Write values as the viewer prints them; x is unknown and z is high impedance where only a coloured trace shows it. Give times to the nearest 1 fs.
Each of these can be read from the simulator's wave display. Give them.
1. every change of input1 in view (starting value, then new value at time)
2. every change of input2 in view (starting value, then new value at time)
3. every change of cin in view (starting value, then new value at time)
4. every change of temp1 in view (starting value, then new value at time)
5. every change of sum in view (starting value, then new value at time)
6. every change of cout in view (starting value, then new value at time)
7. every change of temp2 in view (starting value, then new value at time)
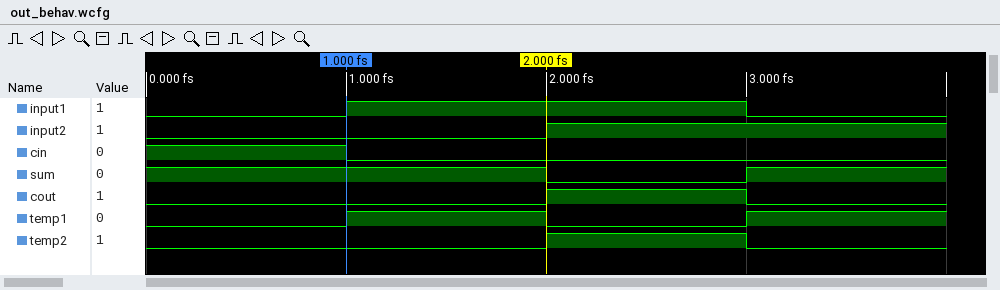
0, 1 at 1 fs, 0 at 3 fs
0, 1 at 2 fs
1, 0 at 1 fs
0, 1 at 1 fs, 0 at 2 fs, 1 at 3 fs
1, 0 at 2 fs, 1 at 3 fs
0, 1 at 2 fs, 0 at 3 fs
0, 1 at 2 fs, 0 at 3 fs
